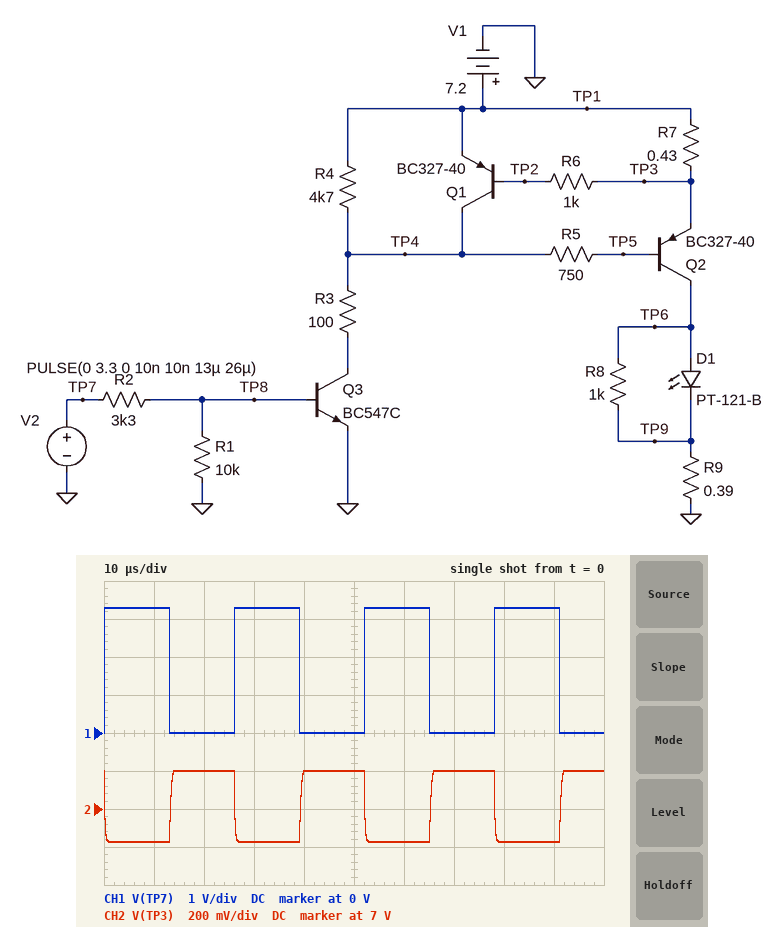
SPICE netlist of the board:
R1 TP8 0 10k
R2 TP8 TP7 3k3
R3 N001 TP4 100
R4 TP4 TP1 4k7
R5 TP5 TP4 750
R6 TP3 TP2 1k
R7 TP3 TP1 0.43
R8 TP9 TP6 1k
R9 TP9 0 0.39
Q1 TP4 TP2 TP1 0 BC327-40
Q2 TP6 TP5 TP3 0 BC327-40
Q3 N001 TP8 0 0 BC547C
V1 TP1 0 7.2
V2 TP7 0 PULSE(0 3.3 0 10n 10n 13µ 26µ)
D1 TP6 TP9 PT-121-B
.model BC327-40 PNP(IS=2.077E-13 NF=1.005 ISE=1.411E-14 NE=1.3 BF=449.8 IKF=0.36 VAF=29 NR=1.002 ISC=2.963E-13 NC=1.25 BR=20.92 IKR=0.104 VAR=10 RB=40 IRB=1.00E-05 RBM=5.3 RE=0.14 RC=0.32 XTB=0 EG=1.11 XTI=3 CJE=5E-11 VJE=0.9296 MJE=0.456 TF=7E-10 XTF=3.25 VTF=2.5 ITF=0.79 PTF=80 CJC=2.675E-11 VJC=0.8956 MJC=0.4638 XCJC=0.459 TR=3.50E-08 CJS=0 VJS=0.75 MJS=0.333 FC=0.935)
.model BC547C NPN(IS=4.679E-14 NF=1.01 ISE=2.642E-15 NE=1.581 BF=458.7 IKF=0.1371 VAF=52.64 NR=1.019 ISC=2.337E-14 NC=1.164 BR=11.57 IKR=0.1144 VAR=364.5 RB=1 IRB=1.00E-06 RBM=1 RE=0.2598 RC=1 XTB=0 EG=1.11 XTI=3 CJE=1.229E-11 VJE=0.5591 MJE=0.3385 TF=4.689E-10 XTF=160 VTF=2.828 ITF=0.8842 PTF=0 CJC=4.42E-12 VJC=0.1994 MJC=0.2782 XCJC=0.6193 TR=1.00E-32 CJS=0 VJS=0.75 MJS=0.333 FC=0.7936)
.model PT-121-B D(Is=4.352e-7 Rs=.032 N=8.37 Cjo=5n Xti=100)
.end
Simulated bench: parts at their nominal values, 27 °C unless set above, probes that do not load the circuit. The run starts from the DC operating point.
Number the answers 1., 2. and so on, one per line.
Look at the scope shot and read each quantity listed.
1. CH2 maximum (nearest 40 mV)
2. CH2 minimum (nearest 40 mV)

1. 7.20 V
2. 6.84 V
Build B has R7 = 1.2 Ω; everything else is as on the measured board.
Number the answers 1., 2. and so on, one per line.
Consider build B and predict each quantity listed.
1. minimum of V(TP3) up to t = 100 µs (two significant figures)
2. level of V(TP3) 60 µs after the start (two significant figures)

1. 6.4 V
2. 6.5 V
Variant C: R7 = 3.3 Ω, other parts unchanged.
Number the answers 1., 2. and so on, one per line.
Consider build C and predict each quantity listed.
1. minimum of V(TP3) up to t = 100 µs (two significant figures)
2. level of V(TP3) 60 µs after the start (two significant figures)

1. 6.0 V
2. 6.4 V
